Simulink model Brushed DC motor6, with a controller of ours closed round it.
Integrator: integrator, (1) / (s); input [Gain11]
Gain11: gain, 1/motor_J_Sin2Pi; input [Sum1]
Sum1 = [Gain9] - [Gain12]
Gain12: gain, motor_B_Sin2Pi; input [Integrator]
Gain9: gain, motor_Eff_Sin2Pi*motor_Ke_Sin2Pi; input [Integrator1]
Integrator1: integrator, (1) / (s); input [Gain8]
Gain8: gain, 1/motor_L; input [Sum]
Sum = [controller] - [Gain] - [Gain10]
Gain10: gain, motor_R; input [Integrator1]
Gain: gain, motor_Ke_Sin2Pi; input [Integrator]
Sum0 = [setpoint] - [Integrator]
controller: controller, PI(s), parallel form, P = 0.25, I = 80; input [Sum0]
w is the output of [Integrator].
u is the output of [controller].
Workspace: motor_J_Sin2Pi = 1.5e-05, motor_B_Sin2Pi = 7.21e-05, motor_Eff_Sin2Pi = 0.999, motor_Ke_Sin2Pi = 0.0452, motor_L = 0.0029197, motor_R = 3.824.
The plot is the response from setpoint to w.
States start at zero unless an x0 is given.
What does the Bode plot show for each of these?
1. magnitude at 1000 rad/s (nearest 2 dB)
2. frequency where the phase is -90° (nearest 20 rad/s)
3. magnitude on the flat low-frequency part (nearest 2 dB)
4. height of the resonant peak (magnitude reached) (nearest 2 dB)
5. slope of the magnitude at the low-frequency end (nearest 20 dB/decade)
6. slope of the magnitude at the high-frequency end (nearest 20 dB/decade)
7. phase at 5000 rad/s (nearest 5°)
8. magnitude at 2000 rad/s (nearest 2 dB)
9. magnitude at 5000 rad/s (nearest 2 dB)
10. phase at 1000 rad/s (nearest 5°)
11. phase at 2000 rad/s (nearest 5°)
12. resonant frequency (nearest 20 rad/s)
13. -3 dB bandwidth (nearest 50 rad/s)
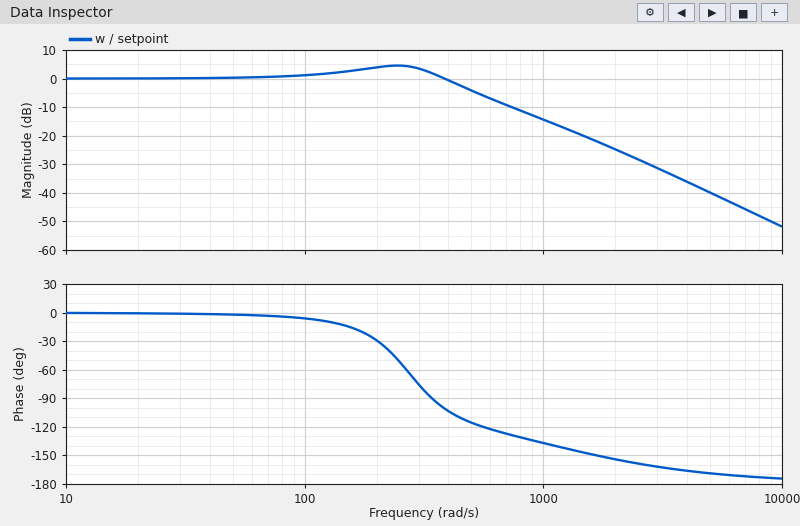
-14 dB
340 rad/s
0 dB
4 dB
0 dB/decade
-40 dB/decade
-170°
-24 dB
-40 dB
-135°
-155°
240 rad/s
450 rad/s
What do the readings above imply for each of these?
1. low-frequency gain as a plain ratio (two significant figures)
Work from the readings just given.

1.0
